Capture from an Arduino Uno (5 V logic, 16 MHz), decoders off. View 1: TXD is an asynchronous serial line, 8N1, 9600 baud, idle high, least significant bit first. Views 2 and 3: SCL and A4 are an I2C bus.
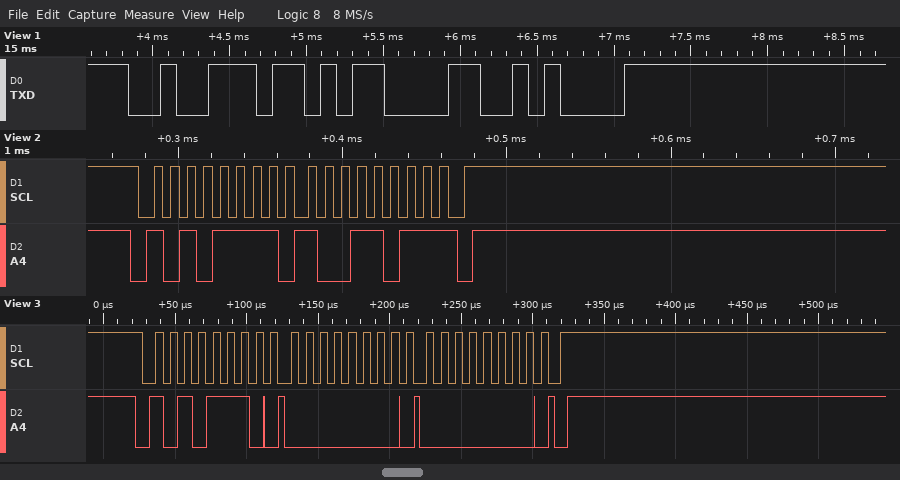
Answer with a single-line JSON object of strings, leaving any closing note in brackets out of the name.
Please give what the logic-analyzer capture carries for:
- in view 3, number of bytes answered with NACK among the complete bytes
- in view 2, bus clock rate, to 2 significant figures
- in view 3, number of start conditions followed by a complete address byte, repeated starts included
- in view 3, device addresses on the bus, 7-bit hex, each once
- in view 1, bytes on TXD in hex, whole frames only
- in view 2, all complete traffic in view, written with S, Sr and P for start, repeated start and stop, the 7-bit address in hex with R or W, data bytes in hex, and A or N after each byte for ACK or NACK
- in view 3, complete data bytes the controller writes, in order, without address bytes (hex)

{"in view 3, number of bytes answered with NACK among the complete bytes": "0", "in view 2, bus clock rate, to 2 significant figures": "100 kHz", "in view 3, number of start conditions followed by a complete address byte, repeated starts included": "1", "in view 3, device addresses on the bus, 7-bit hex, each once": "0x57", "in view 1, bytes on TXD in hex, whole frames only": "72 0D 0A", "in view 2, all complete traffic in view, written with S, Sr and P for start, repeated start and stop, the 7-bit address in hex with R or W, data bytes in hex, and A or N after each byte for ACK or NACK": "S 57R A 9B N P", "in view 3, complete data bytes the controller writes, in order, without address bytes": "00 00"}
